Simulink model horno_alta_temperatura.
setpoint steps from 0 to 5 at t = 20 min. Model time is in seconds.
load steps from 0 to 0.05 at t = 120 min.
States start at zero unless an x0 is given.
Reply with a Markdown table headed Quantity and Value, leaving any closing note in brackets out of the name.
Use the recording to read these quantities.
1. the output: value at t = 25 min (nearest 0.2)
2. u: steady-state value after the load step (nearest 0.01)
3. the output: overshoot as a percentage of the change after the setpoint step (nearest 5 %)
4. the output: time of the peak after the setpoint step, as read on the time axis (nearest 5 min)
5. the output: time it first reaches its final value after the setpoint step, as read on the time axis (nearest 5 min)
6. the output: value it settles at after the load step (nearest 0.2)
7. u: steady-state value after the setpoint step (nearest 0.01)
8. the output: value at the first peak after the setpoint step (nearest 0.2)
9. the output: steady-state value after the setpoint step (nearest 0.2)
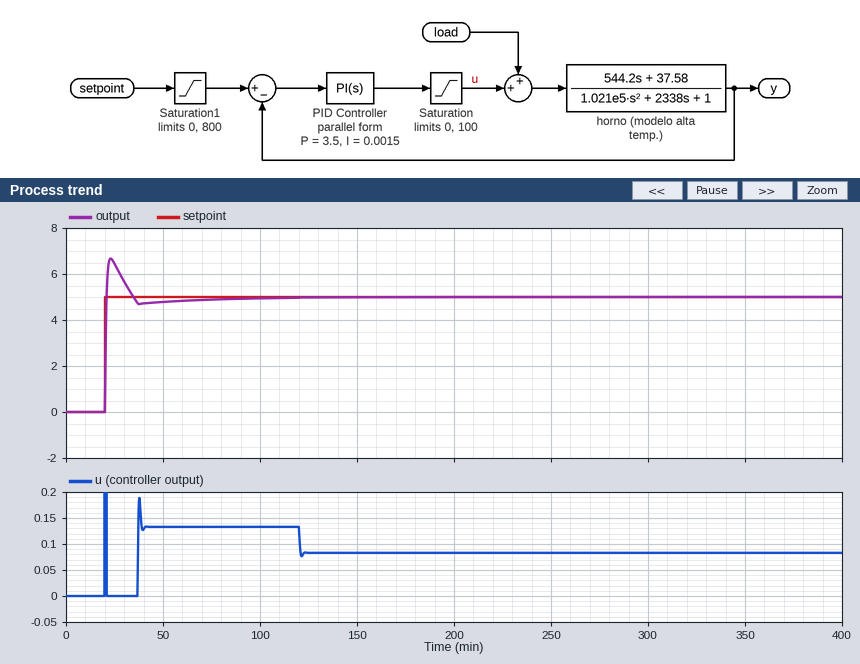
| Quantity | Value |
|---|---|
| the output: value at t = 25 min | 6.4 |
| u: steady-state value after the load step | 0.08 |
| the output: overshoot as a percentage of the change after the setpoint step | 35 % |
| the output: time of the peak after the setpoint step, as read on the time axis | 25 min |
| the output: time it first reaches its final value after the setpoint step, as read on the time axis | 20 min |
| the output: value it settles at after the load step | 5.0 |
| u: steady-state value after the setpoint step | 0.13 |
| the output: value at the first peak after the setpoint step | 6.6 |
| the output: steady-state value after the setpoint step | 5.0 |
